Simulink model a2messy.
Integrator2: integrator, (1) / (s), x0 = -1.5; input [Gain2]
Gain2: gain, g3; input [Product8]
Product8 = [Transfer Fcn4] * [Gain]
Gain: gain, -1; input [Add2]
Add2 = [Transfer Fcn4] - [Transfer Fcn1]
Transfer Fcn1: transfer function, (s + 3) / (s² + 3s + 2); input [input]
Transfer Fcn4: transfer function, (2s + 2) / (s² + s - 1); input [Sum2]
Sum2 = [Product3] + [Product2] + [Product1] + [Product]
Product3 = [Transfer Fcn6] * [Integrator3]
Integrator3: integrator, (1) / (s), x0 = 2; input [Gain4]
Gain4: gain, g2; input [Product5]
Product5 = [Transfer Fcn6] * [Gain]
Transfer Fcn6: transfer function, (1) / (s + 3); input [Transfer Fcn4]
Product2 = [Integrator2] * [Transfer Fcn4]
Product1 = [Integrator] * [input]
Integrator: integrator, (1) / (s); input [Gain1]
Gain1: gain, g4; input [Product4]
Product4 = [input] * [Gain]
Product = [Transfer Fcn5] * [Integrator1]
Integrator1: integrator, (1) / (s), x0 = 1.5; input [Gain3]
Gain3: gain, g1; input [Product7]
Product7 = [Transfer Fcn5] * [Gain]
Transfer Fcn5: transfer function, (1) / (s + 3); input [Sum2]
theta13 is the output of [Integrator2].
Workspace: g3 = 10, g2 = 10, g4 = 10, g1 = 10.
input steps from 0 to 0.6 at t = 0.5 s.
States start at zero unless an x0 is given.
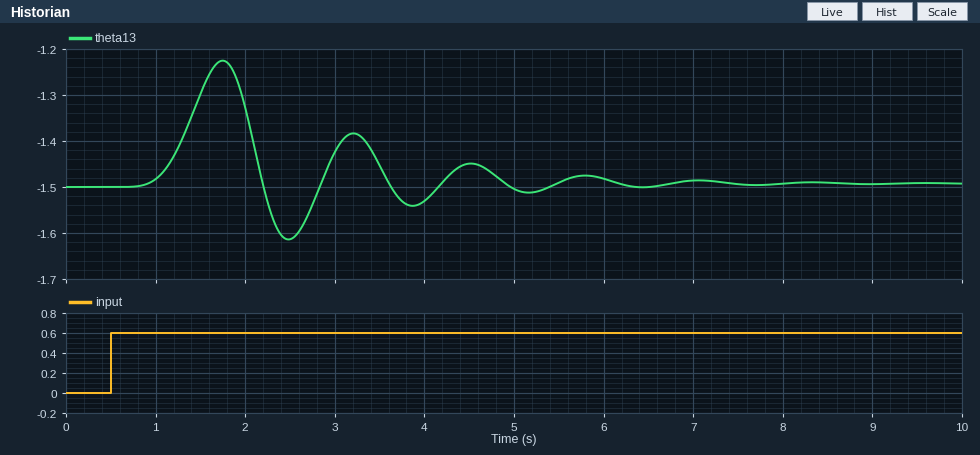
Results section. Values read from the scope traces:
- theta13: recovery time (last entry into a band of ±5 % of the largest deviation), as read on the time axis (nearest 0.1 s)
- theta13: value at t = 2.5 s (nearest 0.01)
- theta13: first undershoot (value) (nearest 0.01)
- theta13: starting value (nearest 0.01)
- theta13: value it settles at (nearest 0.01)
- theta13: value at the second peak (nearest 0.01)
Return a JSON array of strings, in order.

["5.9 s", "-1.61", "-1.61", "-1.50", "-1.49", "-1.38"]
